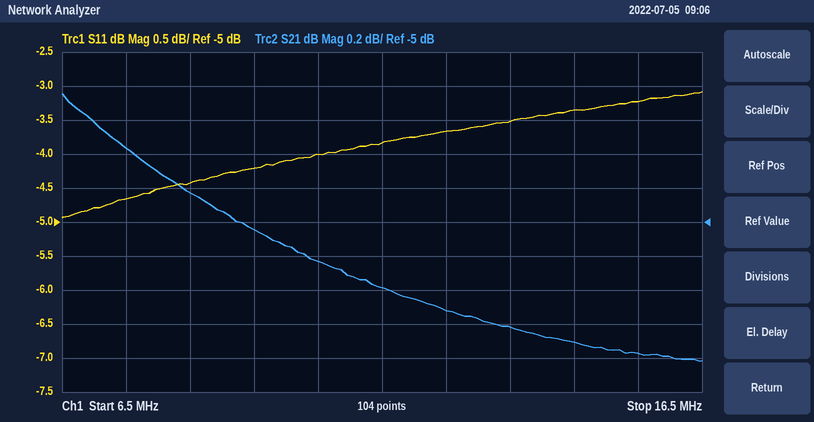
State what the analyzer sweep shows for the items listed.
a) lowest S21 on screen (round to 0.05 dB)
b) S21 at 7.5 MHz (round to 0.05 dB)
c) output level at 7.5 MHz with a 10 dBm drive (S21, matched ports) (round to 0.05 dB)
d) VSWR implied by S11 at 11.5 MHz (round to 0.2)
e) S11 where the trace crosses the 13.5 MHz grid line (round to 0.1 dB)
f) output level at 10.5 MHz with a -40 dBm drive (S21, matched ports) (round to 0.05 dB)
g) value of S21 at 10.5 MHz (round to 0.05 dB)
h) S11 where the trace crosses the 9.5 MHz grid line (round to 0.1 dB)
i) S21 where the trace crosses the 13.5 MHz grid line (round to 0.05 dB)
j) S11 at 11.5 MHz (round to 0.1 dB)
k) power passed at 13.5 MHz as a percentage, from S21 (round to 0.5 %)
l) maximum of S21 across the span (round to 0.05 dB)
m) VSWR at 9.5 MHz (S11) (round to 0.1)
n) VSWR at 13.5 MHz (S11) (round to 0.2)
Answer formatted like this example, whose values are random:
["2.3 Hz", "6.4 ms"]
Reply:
["-5.80 dB", "-4.55 dB", "5.45 dBm", "4.6", "-3.5 dB", "-45.25 dBm", "-5.25 dB", "-4.2 dB", "-5.60 dB", "-3.8 dB", "27.5 %", "-4.25 dB", "4.2", "5.0"]
